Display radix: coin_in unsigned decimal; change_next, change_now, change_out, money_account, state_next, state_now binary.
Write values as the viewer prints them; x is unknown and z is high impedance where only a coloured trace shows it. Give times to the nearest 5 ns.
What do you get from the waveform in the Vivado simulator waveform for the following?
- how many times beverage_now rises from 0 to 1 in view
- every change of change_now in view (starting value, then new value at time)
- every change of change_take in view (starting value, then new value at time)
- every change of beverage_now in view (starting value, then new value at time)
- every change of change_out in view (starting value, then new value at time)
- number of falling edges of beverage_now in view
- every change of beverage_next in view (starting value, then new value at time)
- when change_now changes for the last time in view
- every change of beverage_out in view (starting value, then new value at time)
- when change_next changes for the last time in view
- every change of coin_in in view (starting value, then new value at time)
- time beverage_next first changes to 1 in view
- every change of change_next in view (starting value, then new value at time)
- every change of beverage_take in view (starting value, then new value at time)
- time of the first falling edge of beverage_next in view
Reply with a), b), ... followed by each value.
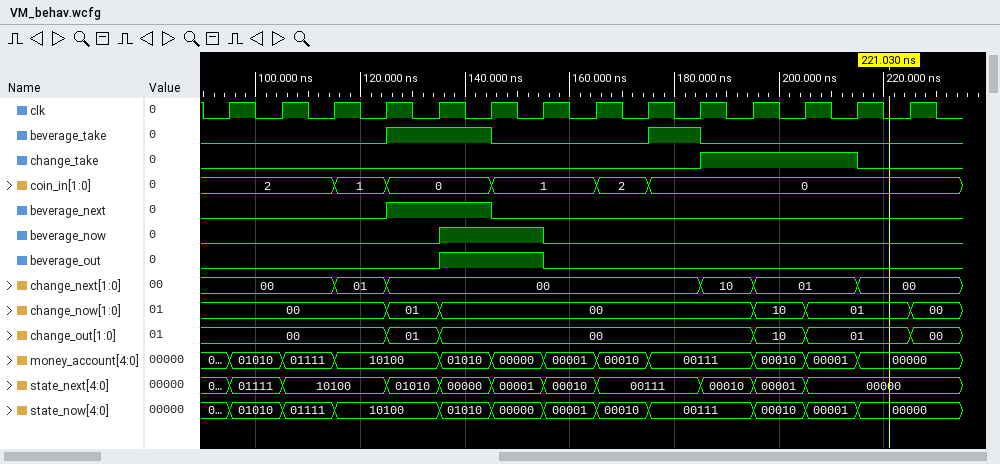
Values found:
a) 1
b) 00, 01 at 125 ns, 00 at 135 ns, 10 at 195 ns, 01 at 205 ns, 00 at 225 ns
c) 0, 1 at 185 ns, 0 at 215 ns
d) 0, 1 at 135 ns, 0 at 155 ns
e) 00, 01 at 125 ns, 00 at 135 ns, 10 at 195 ns, 01 at 205 ns, 00 at 225 ns
f) 1
g) 0, 1 at 125 ns, 0 at 145 ns
h) 225 ns
i) 0, 1 at 135 ns, 0 at 155 ns
j) 215 ns
k) 2, 1 at 115 ns, 0 at 125 ns, 1 at 145 ns, 2 at 165 ns, 0 at 175 ns
l) 125 ns
m) 00, 01 at 115 ns, 00 at 125 ns, 10 at 185 ns, 01 at 195 ns, 00 at 215 ns
n) 0, 1 at 125 ns, 0 at 145 ns, 1 at 175 ns, 0 at 185 ns
o) 145 ns
